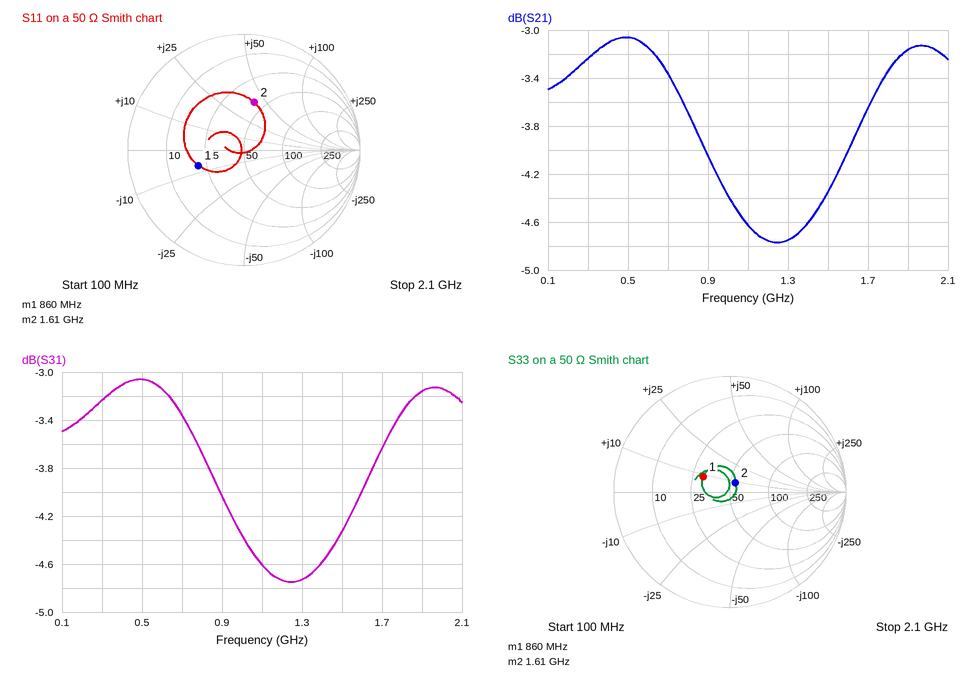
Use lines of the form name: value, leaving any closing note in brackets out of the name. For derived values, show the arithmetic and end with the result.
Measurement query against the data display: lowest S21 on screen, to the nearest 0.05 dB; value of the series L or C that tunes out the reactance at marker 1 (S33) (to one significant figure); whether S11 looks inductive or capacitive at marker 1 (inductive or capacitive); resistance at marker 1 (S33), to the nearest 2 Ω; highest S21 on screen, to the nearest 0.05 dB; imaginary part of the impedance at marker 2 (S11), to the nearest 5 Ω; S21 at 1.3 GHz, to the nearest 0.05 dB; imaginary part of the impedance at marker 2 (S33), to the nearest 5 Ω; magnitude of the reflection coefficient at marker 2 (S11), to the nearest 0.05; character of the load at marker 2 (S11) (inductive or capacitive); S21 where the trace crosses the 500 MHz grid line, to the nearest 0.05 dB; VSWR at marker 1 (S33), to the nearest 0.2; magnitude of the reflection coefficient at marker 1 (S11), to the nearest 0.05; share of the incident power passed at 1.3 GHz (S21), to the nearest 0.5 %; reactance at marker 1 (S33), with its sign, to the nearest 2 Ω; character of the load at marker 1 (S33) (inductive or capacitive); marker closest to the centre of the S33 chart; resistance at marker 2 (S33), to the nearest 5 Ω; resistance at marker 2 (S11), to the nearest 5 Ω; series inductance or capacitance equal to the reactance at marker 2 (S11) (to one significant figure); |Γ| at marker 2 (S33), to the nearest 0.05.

lowest S21 on screen, to the nearest 0.05 dB: -4.75 dB
value of the series L or C that tunes out the reactance at marker 1 (S33): C = 1/(2π × 860 MHz × 8 Ω) ≈ 23.1 pF, so 20 pF to one significant figure
whether S11 looks inductive or capacitive at marker 1: capacitive
resistance at marker 1 (S33), to the nearest 2 Ω: 30 Ω
highest S21 on screen, to the nearest 0.05 dB: -3.05 dB
imaginary part of the impedance at marker 2 (S11), to the nearest 5 Ω: +40 Ω
S21 at 1.3 GHz, to the nearest 0.05 dB: -4.75 dB
imaginary part of the impedance at marker 2 (S33), to the nearest 5 Ω: +10 Ω
magnitude of the reflection coefficient at marker 2 (S11), to the nearest 0.05: 0.40
character of the load at marker 2 (S11): inductive
S21 where the trace crosses the 500 MHz grid line, to the nearest 0.05 dB: -3.05 dB
VSWR at marker 1 (S33), to the nearest 0.2: 1.8
magnitude of the reflection coefficient at marker 1 (S11), to the nearest 0.05: 0.40
share of the incident power passed at 1.3 GHz (S21), to the nearest 0.5 %: 10^(-4.75/10) ≈ 33.5 %
reactance at marker 1 (S33), with its sign, to the nearest 2 Ω: +8 Ω
character of the load at marker 1 (S33): inductive
marker closest to the centre of the S33 chart: marker 2
resistance at marker 2 (S33), to the nearest 5 Ω: 55 Ω
resistance at marker 2 (S11), to the nearest 5 Ω: 40 Ω
series inductance or capacitance equal to the reactance at marker 2 (S11): L = 40 Ω/(2π × 1.61 GHz) ≈ 4 nH
|Γ| at marker 2 (S33), to the nearest 0.05: 0.10
